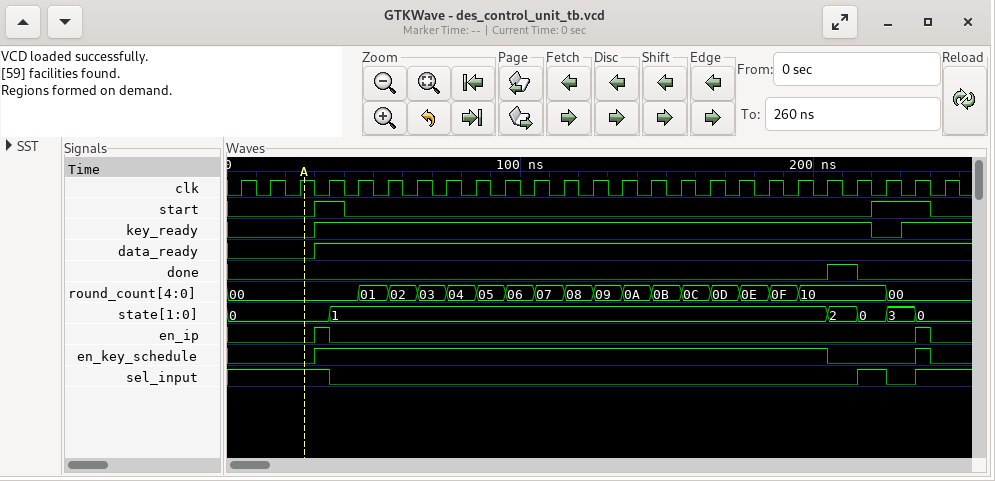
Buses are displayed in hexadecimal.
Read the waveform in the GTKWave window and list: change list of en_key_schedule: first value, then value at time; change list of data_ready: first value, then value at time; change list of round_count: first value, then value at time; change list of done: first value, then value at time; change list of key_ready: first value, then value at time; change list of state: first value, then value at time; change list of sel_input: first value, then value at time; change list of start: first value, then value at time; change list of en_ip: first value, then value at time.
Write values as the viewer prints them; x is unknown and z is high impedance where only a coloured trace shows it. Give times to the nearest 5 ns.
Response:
0, 1 at 30 ns, 0 at 205 ns, 1 at 235 ns, 0 at 240 ns
0, 1 at 30 ns
00, 01 at 45 ns, 02 at 55 ns, 03 at 65 ns, 04 at 75 ns, 05 at 85 ns, 06 at 95 ns, 07 at 105 ns, 08 at 115 ns, 09 at 125 ns, 0A at 135 ns, 0B at 145 ns, 0C at 155 ns, 0D at 165 ns, 0E at 175 ns, 0F at 185 ns, 10 at 195 ns, 00 at 225 ns
0, 1 at 205 ns, 0 at 215 ns
0, 1 at 30 ns, 0 at 220 ns, 1 at 230 ns
0, 1 at 35 ns, 2 at 205 ns, 0 at 215 ns, 3 at 225 ns, 0 at 235 ns
1, 0 at 35 ns, 1 at 215 ns, 0 at 225 ns, 1 at 235 ns
0, 1 at 30 ns, 0 at 40 ns, 1 at 220 ns, 0 at 240 ns
0, 1 at 30 ns, 0 at 35 ns, 1 at 235 ns, 0 at 240 ns
